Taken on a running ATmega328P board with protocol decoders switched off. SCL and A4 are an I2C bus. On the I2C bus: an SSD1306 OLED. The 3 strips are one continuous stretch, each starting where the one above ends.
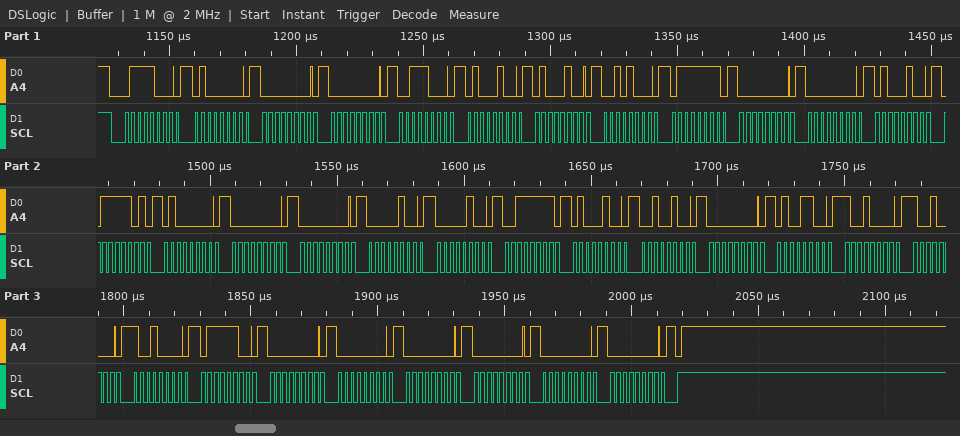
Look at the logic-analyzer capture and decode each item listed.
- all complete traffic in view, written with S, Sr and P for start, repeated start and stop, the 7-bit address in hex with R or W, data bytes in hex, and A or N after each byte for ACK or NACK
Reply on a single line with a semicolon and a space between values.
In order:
S 3CW A 40 A 00 A 00 A 38 A 44 A 44 A 28 A 7F A 00 A 00 A 44 A 7D A 40 A 00 A 00 A 04 A 04 A 3F A 44 A 24 A 00 A 4C A 90 A 90 A 90 A 7C A 00 A 00 A 00 A 00 A 00 A 00 A P
